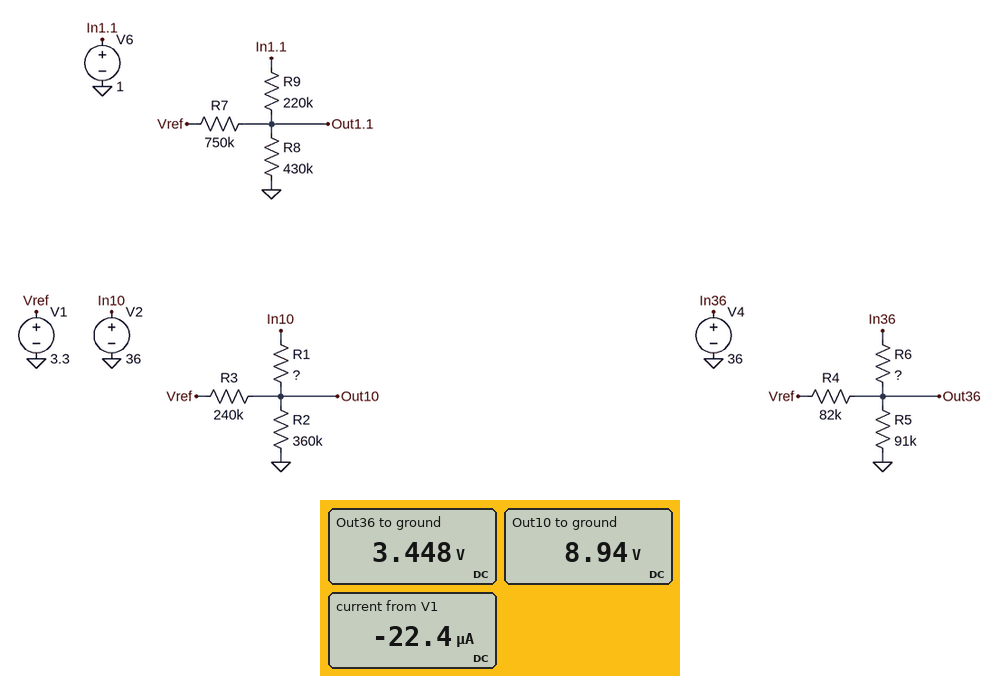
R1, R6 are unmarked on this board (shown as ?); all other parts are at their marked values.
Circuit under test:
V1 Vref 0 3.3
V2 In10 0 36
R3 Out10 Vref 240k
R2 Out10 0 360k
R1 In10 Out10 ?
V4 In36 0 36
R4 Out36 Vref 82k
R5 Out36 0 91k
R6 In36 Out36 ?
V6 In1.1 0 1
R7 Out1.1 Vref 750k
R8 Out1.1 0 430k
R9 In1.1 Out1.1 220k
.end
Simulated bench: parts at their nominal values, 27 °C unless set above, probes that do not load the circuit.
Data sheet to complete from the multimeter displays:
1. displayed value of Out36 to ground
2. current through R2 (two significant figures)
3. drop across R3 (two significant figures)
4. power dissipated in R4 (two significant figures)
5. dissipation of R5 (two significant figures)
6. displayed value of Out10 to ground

3.448 V
25 µA
5.6 V
270 nW
130 µW
8.94 V
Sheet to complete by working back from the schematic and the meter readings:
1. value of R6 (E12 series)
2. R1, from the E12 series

820 kΩ
560 kΩ
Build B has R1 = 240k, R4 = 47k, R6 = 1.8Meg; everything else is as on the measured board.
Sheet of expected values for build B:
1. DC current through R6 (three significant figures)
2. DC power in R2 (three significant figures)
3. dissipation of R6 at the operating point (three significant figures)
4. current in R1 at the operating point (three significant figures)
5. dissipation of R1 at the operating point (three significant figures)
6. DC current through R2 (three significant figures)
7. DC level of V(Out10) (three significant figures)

18.5 µA
603 µW
614 µW
88.6 µA
1.88 mW
40.9 µA
14.7 V
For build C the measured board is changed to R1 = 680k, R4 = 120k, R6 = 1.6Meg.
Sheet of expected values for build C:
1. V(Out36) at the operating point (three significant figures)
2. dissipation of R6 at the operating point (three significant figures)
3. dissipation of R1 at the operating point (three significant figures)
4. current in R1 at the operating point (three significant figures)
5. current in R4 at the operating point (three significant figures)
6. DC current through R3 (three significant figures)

2.51 V
701 µW
1.16 mW
41.3 µA
6.61 µA
19.3 µA
